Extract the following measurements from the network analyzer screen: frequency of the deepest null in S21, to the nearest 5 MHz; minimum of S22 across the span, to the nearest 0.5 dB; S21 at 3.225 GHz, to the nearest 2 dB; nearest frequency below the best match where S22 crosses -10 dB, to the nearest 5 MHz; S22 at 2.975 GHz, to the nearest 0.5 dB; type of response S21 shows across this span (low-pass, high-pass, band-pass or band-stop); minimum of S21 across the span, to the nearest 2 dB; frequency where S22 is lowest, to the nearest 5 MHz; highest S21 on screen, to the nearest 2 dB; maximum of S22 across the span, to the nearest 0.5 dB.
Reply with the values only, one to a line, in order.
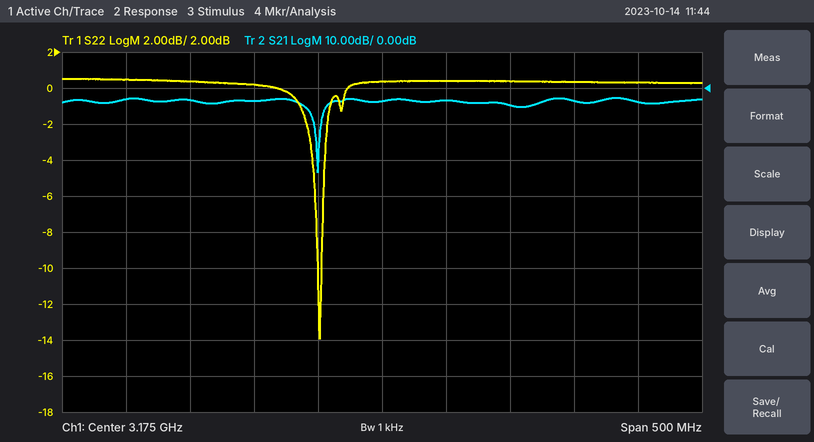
3.125 GHz
-14.0 dB
-4 dB
3.125 GHz
0.5 dB
band-stop
-24 dB
3.125 GHz
-2 dB
0.5 dB
